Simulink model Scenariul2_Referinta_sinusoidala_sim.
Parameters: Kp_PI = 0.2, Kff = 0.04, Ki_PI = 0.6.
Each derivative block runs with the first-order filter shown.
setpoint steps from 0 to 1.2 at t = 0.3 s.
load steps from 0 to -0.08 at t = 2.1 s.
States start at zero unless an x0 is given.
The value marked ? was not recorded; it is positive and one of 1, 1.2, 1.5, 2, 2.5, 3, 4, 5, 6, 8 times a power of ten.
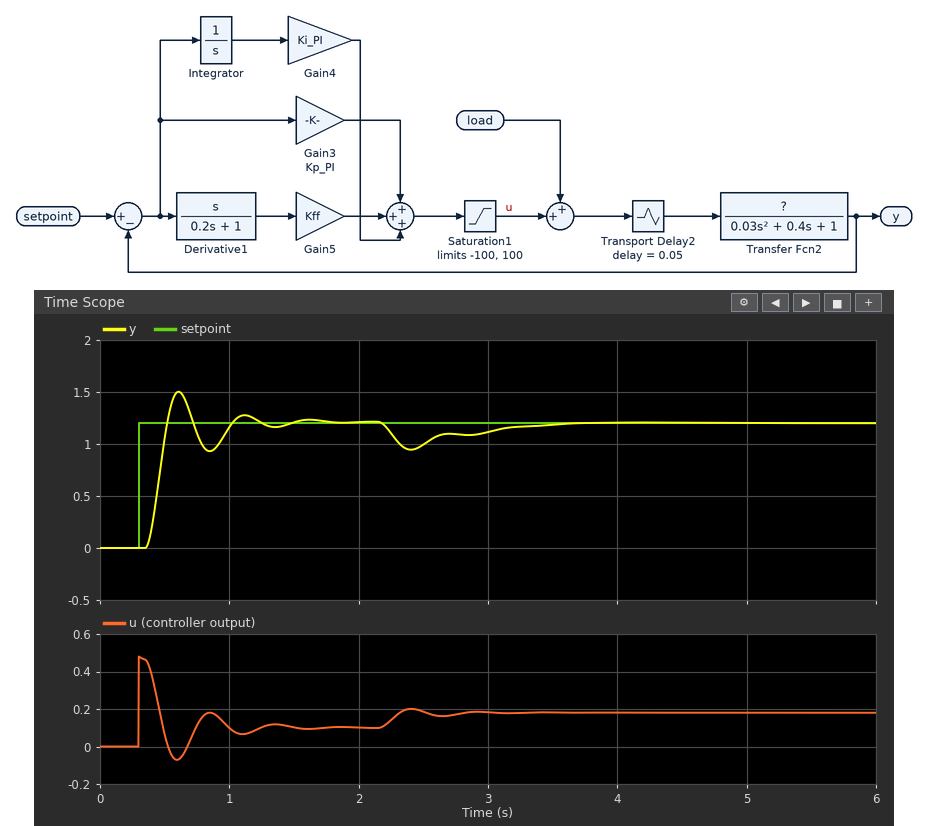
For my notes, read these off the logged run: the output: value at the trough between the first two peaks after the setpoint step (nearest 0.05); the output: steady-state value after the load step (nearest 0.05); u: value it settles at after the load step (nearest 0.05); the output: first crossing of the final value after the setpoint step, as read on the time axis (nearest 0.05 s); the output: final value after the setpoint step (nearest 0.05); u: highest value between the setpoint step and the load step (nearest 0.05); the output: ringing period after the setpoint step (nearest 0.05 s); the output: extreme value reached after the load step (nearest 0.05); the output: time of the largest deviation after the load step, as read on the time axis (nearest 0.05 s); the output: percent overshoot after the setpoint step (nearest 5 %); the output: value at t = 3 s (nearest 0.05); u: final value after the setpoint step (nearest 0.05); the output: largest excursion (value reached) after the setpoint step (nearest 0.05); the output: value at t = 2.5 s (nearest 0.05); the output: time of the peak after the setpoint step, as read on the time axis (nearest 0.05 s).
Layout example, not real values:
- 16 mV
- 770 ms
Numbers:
- 0.95
- 1.20
- 0.20
- 0.50 s
- 1.20
- 0.50
- 0.50 s
- 0.95
- 2.40 s
- 25 %
- 1.10
- 0.10
- 1.50
- 1.00
- 0.60 s
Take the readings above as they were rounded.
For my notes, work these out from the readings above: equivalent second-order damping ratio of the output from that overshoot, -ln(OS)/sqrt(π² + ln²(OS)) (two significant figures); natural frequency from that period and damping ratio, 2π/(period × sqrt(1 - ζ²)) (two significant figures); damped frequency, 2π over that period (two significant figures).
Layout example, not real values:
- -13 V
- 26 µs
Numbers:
- 0.40
- 14 rad/s
- 13 rad/s
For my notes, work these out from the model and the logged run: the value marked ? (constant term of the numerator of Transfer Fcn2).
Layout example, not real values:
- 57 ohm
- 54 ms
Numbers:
- 12
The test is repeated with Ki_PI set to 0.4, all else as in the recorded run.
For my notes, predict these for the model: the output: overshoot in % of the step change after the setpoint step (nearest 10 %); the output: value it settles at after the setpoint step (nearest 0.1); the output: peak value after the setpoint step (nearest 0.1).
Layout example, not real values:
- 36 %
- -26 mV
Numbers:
- 20 %
- 1.2
- 1.4
